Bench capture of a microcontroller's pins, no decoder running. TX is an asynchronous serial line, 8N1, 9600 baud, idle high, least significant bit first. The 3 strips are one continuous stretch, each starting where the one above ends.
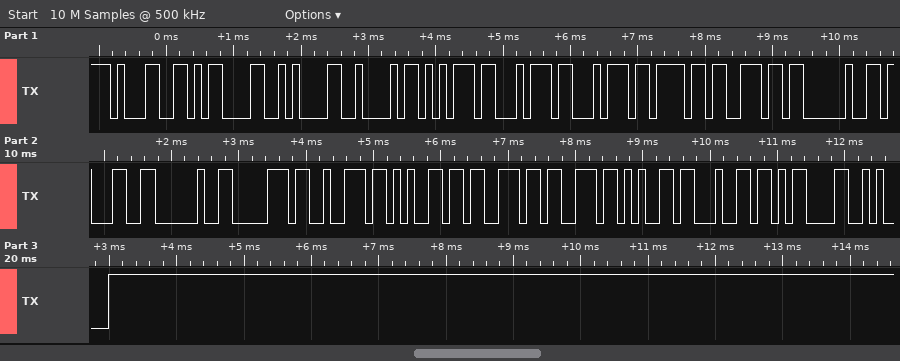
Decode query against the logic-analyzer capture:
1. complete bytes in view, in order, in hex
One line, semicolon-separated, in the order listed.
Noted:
31 0D 0A 42 75 74 74 6F 6E 20 31 20 70 72 65 73 73 65 64 0D 0A
